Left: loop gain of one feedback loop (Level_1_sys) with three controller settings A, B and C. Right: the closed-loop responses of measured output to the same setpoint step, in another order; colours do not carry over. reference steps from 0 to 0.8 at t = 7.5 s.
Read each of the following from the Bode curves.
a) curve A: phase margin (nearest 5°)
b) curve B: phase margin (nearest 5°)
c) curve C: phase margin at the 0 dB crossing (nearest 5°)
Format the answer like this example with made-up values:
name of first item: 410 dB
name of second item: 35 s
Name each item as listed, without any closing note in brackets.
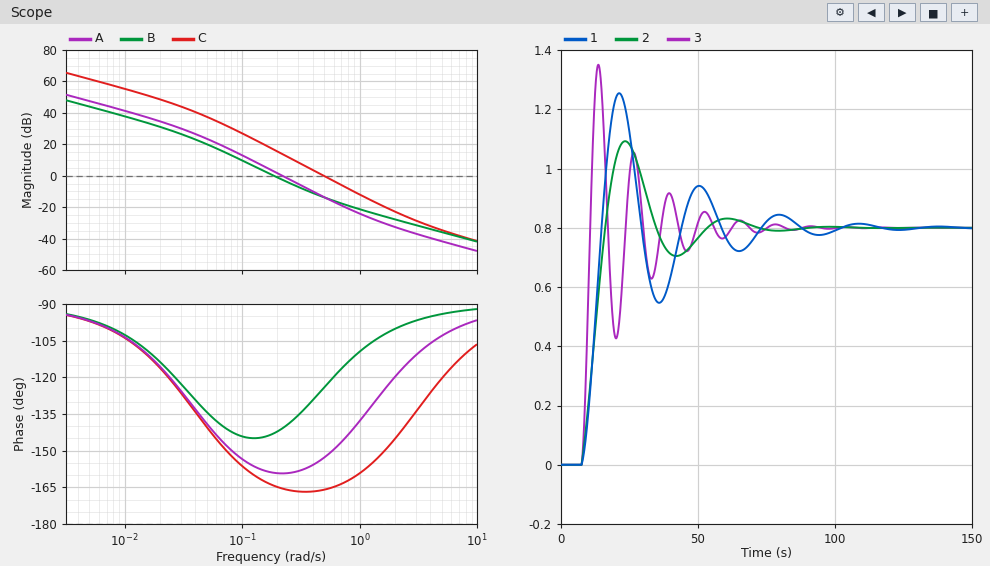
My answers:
curve A: phase margin: 20°
curve B: phase margin: 35°
curve C: phase margin at the 0 dB crossing: 15°
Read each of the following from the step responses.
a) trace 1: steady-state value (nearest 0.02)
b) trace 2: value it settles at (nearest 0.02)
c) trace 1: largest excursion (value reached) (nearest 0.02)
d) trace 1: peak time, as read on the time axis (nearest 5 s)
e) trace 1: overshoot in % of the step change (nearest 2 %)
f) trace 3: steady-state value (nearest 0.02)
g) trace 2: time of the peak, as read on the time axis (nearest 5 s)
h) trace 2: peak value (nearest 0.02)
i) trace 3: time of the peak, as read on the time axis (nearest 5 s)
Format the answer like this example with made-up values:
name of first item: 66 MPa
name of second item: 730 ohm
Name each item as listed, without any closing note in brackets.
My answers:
trace 1: steady-state value: 0.80
trace 2: value it settles at: 0.80
trace 1: largest excursion (value reached): 1.26
trace 1: peak time, as read on the time axis: 20 s
trace 1: overshoot in % of the step change: 56 %
trace 3: steady-state value: 0.80
trace 2: time of the peak, as read on the time axis: 25 s
trace 2: peak value: 1.10
trace 3: time of the peak, as read on the time axis: 15 s
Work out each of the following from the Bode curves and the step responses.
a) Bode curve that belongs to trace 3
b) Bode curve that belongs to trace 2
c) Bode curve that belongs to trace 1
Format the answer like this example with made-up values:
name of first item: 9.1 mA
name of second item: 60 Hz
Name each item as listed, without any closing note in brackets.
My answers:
Bode curve that belongs to trace 3: C
Bode curve that belongs to trace 2: B
Bode curve that belongs to trace 1: A
